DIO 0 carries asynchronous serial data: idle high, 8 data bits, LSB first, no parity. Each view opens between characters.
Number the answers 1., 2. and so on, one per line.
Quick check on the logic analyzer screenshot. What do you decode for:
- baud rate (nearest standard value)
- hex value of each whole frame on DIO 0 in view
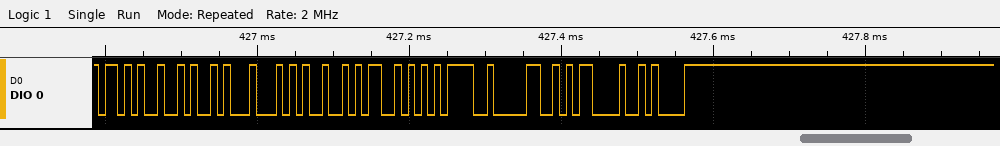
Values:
1. 115200 baud
2. 2B, 4A, 44, 49, 53, 3D, 30, 0D, 0A
